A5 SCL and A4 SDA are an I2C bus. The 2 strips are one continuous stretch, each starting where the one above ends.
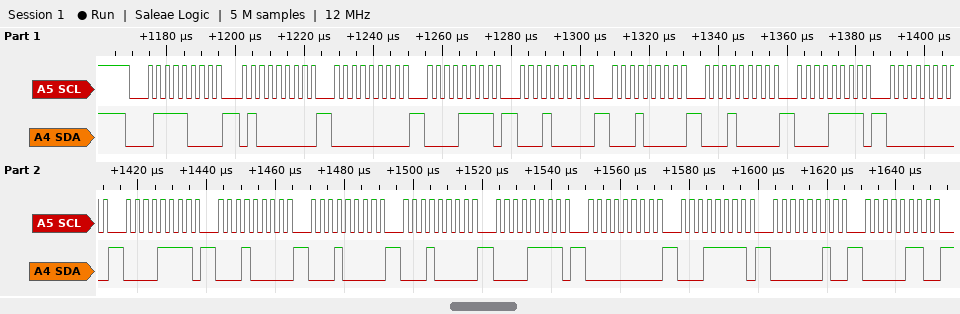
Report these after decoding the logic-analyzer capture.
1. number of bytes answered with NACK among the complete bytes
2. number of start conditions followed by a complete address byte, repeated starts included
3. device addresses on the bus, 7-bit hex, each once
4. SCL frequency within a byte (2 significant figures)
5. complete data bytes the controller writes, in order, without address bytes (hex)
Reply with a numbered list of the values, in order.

1. 0
2. 1
3. 0x3C
4. 400 kHz
5. 40 00 0F 10 10 10 0F 00 0F 10 10 10 0F 00 1F 02 06
